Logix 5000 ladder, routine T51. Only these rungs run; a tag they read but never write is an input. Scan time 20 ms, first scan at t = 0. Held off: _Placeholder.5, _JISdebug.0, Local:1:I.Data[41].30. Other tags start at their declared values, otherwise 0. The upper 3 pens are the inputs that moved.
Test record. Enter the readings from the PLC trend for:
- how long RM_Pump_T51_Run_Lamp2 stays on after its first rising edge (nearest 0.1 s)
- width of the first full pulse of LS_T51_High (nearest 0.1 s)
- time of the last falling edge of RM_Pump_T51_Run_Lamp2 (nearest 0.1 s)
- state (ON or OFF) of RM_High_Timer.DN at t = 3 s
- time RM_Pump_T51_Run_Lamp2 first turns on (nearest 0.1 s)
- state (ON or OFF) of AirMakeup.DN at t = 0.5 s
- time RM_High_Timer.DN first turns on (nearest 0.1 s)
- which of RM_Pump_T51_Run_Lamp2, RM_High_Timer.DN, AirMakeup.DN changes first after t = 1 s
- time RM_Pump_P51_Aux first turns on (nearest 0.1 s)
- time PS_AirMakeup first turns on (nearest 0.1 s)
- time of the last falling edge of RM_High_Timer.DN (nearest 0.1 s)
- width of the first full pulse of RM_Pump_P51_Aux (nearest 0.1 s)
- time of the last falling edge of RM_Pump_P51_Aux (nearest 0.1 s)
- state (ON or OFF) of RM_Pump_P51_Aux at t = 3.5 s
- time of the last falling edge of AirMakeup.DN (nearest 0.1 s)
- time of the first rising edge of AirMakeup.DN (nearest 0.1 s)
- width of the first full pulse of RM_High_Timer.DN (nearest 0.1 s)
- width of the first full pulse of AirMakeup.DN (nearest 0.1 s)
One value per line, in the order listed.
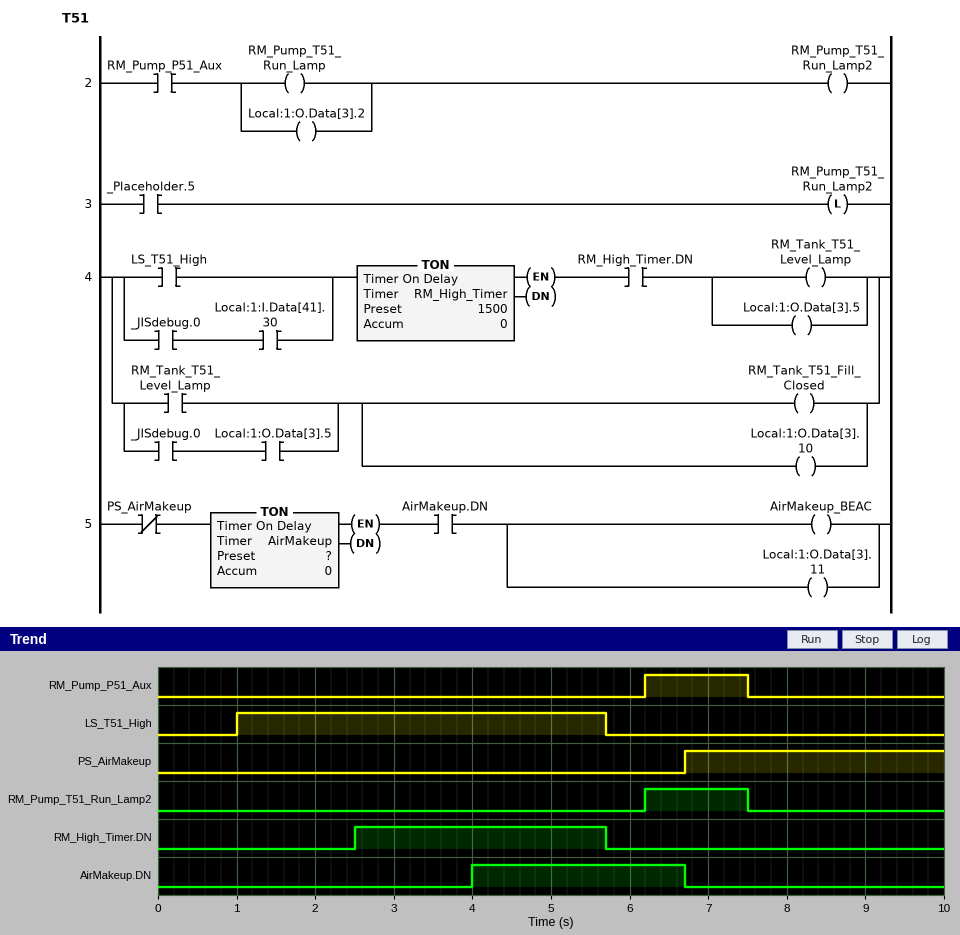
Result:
1.3 s
4.7 s
7.5 s
ON
6.2 s
OFF
2.5 s
RM_High_Timer.DN
6.2 s
6.7 s
5.7 s
1.3 s
7.5 s
OFF
6.7 s
4.0 s
3.2 s
2.7 s
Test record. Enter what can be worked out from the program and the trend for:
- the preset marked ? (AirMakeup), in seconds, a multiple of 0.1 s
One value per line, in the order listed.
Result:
4.0 s
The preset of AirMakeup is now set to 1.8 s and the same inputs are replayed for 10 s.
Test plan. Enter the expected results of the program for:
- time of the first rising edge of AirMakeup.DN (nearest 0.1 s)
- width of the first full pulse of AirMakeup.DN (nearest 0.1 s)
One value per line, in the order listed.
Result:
1.8 s
4.9 s
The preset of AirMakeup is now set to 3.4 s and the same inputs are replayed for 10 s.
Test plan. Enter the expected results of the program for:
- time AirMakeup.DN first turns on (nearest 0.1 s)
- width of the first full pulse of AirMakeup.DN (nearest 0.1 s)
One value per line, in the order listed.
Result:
3.4 s
3.3 s
